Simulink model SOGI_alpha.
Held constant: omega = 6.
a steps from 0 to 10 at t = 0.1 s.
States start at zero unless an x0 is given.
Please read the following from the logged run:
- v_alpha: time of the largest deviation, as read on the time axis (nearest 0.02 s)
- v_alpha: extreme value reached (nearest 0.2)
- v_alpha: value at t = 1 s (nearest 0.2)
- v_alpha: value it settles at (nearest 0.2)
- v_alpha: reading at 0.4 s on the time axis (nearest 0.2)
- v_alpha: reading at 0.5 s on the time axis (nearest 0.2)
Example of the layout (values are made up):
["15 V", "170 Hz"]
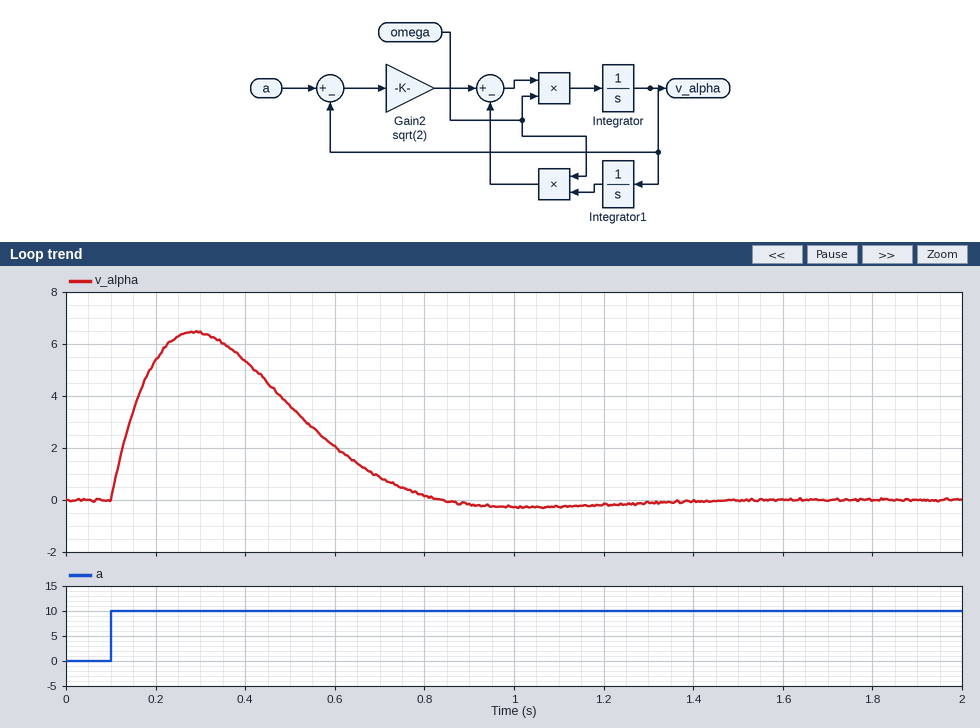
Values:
["0.28 s", "6.4", "-0.2", "0.0", "5.4", "3.6"]
